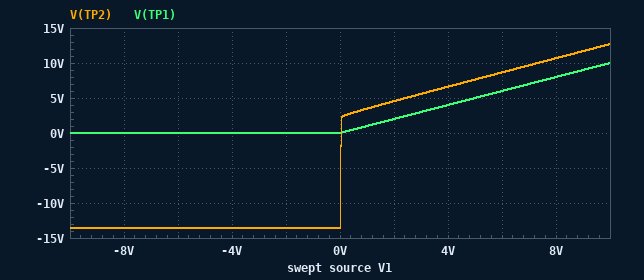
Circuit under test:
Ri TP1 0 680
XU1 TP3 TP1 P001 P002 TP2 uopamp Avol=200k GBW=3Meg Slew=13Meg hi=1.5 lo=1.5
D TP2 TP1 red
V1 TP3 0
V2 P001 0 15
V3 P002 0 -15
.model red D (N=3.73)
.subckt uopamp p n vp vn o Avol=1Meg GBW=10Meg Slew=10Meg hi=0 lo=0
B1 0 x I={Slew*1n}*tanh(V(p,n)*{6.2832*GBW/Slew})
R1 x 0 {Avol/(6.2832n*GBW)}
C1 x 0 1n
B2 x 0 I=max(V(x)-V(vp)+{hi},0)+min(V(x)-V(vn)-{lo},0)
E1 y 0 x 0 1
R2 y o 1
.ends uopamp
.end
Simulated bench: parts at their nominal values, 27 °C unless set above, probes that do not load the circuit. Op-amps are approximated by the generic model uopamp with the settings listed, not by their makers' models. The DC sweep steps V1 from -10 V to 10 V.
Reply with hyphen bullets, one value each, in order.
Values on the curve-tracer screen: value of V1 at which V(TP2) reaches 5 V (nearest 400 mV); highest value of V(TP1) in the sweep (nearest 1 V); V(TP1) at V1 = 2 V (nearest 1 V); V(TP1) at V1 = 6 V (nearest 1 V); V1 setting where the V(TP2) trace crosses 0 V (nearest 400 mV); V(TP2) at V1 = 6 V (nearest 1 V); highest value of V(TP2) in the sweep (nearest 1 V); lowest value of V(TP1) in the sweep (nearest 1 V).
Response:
- 2.4 V
- 10 V
- 2 V
- 6 V
- 0 V
- 9 V
- 13 V
- 0 V
